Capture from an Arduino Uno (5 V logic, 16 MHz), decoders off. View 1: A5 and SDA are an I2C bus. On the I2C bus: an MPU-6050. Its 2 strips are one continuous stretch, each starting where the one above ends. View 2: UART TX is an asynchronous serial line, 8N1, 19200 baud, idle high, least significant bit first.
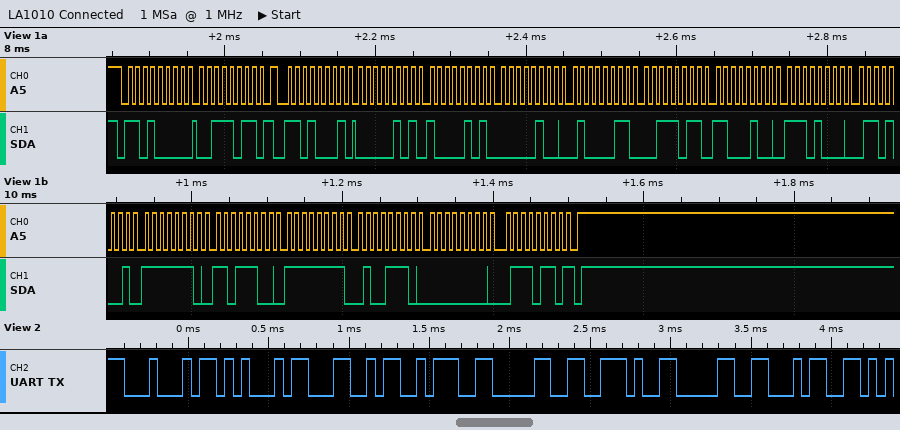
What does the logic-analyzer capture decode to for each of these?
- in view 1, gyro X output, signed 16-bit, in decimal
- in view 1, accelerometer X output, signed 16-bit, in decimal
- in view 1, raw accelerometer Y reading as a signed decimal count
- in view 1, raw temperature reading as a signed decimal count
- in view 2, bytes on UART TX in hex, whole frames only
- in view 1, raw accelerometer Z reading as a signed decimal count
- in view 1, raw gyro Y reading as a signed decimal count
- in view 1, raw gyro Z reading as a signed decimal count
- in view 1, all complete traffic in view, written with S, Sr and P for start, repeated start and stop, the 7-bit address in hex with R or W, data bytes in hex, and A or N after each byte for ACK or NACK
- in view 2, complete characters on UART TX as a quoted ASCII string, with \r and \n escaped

-292
1413
1091
-6039
44 45 4C 3A 30 2E 30 34
15300
-178
118
S 68W A 3B A Sr 68R A 05 A 85 A 04 A 43 A 3B A C4 A E8 A 69 A FE A DC A FF A 4E A 00 A 76 N P
"DEL:0.04"
